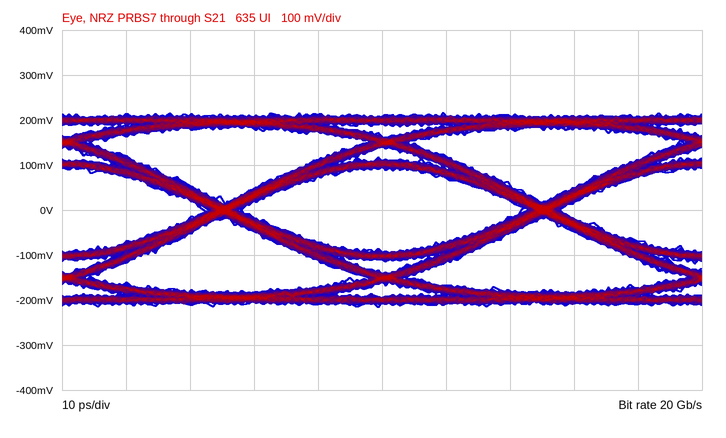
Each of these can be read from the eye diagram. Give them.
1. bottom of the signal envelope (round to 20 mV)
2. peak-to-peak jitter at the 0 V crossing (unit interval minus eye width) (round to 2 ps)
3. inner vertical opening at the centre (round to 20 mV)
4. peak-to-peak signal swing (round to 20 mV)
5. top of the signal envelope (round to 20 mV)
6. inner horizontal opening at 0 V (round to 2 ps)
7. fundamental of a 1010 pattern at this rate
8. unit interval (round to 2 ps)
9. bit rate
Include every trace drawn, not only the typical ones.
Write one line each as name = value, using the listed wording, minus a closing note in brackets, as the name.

bottom of the signal envelope = -220 mV
peak-to-peak jitter at the 0 V crossing (unit interval minus eye width) = 6 ps
inner vertical opening at the centre = 180 mV
peak-to-peak signal swing = 440 mV
top of the signal envelope = 220 mV
inner horizontal opening at 0 V = 44 ps
fundamental of a 1010 pattern at this rate = 10 GHz
unit interval = 50 ps
bit rate = 20 Gb/s
